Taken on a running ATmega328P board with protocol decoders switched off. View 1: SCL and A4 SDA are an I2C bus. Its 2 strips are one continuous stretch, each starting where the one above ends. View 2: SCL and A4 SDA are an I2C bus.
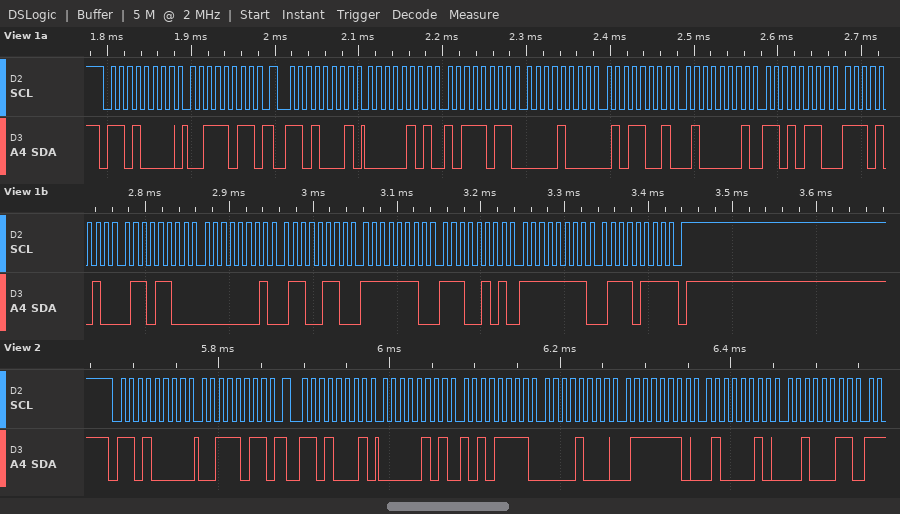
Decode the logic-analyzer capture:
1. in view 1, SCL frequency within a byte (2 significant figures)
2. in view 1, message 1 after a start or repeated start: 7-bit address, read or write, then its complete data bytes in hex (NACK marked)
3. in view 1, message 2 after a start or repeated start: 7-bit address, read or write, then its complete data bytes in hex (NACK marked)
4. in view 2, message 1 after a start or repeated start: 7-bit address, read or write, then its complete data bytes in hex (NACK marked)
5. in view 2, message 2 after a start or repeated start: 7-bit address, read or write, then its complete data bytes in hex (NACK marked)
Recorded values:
100 kHz
0x68 write: 3B
0x68 read: 05 BB 08 59 41 D6 EA 6C 01 66 FE E5 FF 77 NACK
0x68 write: 3B
0x68 read: 05 AF 08 7E 42 23
